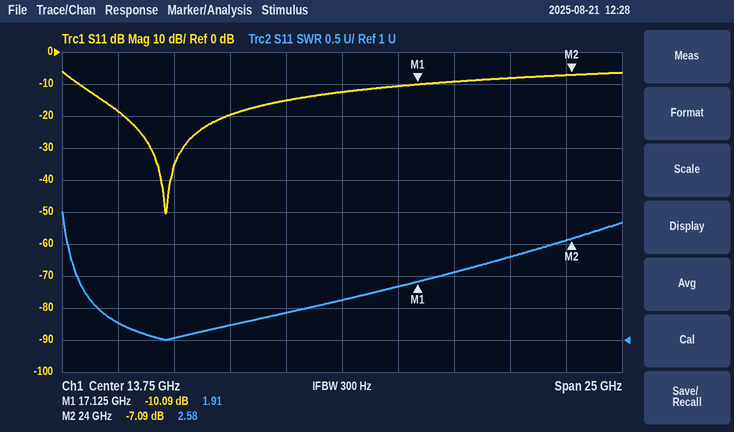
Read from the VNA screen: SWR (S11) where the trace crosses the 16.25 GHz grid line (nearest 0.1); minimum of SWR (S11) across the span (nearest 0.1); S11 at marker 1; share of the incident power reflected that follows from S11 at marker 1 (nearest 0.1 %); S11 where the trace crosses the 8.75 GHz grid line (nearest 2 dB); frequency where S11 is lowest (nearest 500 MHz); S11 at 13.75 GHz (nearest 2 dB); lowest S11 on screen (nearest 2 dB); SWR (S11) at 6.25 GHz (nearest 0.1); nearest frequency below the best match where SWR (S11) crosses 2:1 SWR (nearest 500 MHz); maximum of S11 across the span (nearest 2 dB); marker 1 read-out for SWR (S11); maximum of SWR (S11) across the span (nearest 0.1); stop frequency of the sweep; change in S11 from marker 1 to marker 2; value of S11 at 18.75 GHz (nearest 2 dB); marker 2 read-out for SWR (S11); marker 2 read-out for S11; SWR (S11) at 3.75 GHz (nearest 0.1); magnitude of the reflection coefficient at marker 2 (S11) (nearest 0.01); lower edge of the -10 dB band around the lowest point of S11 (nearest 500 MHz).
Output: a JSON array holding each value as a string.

["1.8", "1.0", "-10.09 dB", "9.8 %", "-20 dB", "6.0 GHz", "-12 dB", "-50 dB", "1.0", "2.0 GHz", "-6 dB", "1.91", "3.0", "26.25 GHz", "3.00 dB", "-10 dB", "2.58", "-7.09 dB", "1.3", "0.44", "2.0 GHz"]
